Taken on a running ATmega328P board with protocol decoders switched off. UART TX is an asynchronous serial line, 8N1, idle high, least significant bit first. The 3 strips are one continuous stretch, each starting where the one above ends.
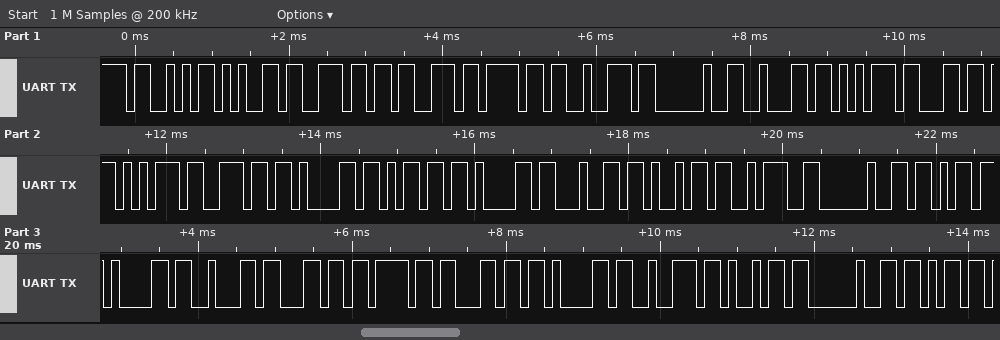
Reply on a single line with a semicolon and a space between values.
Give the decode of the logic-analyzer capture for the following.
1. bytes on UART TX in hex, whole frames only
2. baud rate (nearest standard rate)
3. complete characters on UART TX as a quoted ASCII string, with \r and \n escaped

53 65 6E 73 6F 72 20 62 75 6C 75 6E 61 6D 61 64 69 3A 20 6B 61 62 6C 6F 6C 61 72 69 20 6B; 9600 baud; "Sensor bulunamadi: kablolari k"
